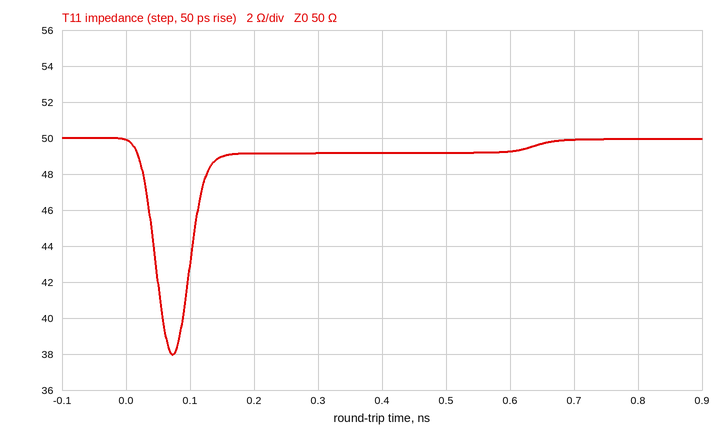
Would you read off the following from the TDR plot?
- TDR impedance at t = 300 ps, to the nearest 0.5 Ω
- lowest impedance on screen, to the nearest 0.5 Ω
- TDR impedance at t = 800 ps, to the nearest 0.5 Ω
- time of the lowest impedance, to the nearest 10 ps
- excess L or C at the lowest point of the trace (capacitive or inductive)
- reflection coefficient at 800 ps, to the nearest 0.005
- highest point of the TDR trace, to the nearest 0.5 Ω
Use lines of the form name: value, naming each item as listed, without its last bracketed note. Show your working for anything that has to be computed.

TDR impedance at t = 300 ps, to the nearest 0.5 Ω: 49.0 Ω
lowest impedance on screen, to the nearest 0.5 Ω: 38.0 Ω
TDR impedance at t = 800 ps, to the nearest 0.5 Ω: 50.0 Ω
time of the lowest impedance, to the nearest 10 ps: 70 ps
excess L or C at the lowest point of the trace: capacitive
reflection coefficient at 800 ps, to the nearest 0.005: (50 − 50)/(50 + 50) ≈ 0.000
highest point of the TDR trace, to the nearest 0.5 Ω: 50.0 Ω
